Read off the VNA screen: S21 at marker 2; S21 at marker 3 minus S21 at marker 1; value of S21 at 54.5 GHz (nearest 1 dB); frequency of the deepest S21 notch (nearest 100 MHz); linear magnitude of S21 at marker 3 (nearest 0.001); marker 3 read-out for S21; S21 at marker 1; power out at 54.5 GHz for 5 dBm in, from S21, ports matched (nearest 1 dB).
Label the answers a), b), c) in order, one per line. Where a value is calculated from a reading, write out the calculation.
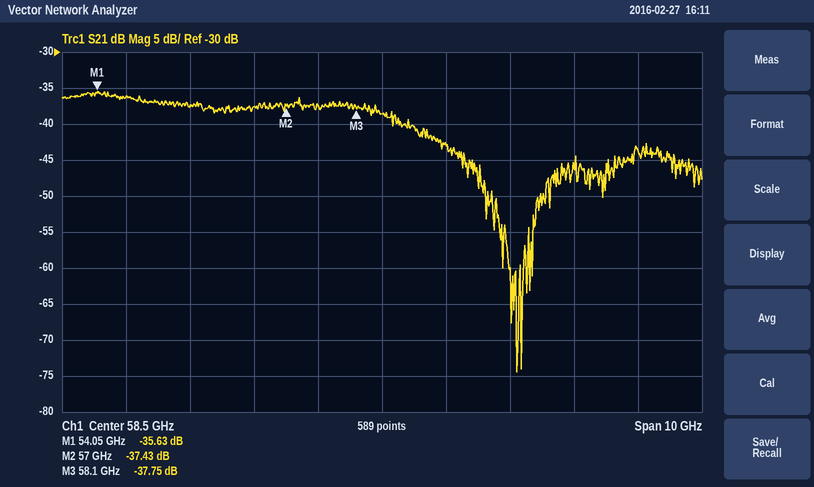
a) -37.43 dB
b) -37.75 − (-35.63) = -2.12 dB
c) -36 dB
d) 60.6 GHz
e) 10^(-37.75/20) ≈ 0.013
f) -37.75 dB
g) -35.63 dB
h) 5 dBm + (-36 dB) = -31 dBm
